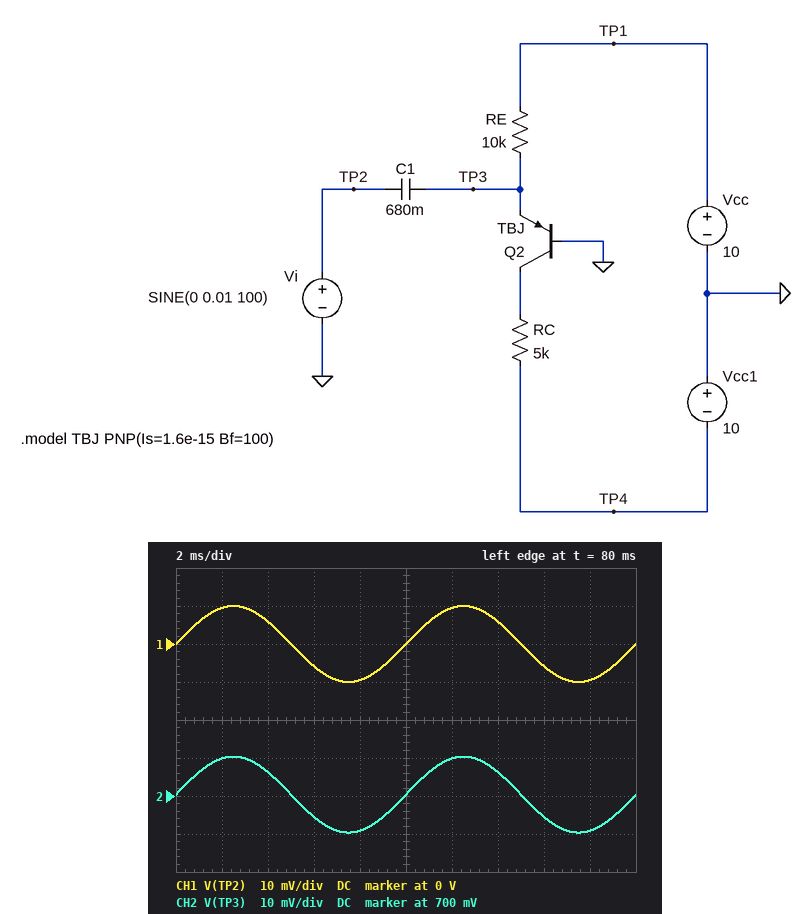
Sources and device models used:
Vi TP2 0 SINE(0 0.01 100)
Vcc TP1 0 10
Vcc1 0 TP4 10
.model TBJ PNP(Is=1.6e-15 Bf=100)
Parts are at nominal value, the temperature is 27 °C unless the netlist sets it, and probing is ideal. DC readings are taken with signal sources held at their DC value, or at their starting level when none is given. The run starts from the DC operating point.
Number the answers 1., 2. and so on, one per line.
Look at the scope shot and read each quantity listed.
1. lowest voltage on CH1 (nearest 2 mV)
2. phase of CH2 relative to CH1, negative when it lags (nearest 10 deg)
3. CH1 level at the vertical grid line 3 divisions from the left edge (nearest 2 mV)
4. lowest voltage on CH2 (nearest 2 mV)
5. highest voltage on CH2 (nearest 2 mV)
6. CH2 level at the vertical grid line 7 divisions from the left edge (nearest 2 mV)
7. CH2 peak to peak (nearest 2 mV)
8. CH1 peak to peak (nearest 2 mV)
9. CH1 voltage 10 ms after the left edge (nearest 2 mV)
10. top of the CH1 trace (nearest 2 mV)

1. -10 mV
2. 0 deg
3. -6 mV
4. 690 mV
5. 710 mV
6. 706 mV
7. 20 mV
8. 20 mV
9. 0 V
10. 10 mV
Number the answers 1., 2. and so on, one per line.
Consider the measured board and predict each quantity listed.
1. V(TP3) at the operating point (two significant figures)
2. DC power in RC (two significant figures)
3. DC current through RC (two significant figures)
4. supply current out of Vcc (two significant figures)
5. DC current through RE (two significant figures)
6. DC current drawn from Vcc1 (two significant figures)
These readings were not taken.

1. 700 mV
2. 4.2 mW
3. 920 µA
4. 930 µA
5. 930 µA
6. 920 µA
